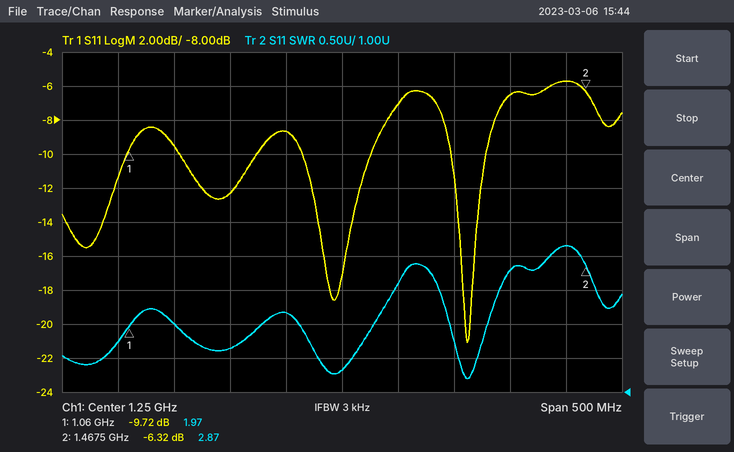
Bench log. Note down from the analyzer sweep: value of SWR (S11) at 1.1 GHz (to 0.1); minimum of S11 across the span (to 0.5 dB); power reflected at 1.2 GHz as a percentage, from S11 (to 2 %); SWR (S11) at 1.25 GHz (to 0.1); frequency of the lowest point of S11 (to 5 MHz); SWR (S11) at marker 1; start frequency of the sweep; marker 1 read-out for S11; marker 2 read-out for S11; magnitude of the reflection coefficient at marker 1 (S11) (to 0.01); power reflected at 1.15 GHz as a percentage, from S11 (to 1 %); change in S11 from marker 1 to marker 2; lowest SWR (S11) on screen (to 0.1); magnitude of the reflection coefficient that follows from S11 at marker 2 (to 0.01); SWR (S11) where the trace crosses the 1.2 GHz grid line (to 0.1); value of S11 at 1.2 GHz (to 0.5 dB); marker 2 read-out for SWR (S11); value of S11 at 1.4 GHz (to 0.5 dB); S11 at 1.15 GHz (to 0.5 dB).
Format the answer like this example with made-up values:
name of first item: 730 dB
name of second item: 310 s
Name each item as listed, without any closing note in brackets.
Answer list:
value of SWR (S11) at 1.1 GHz: 2.0
minimum of S11 across the span: -21.0 dB
power reflected at 1.2 GHz as a percentage, from S11: 14 %
SWR (S11) at 1.25 GHz: 1.3
frequency of the lowest point of S11: 1.360 GHz
SWR (S11) at marker 1: 1.97
start frequency of the sweep: 1 GHz
marker 1 read-out for S11: -9.72 dB
marker 2 read-out for S11: -6.32 dB
magnitude of the reflection coefficient at marker 1 (S11): 0.33
power reflected at 1.15 GHz as a percentage, from S11: 6 %
change in S11 from marker 1 to marker 2: 3.40 dB
lowest SWR (S11) on screen: 1.2
magnitude of the reflection coefficient that follows from S11 at marker 2: 0.48
SWR (S11) where the trace crosses the 1.2 GHz grid line: 2.2
value of S11 at 1.2 GHz: -8.5 dB
marker 2 read-out for SWR: 2.87
value of S11 at 1.4 GHz: -6.5 dB
S11 at 1.15 GHz: -12.5 dB
